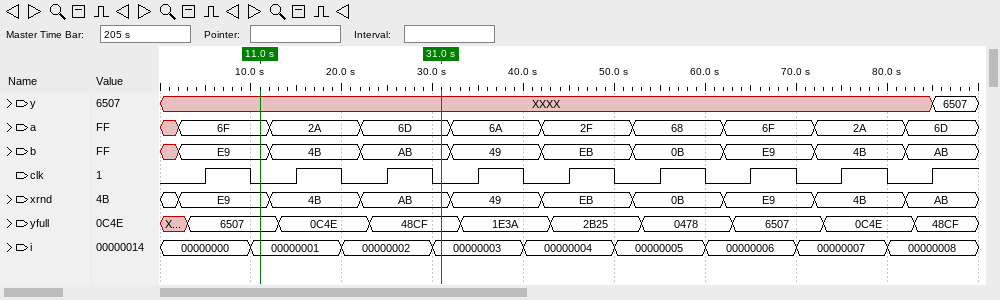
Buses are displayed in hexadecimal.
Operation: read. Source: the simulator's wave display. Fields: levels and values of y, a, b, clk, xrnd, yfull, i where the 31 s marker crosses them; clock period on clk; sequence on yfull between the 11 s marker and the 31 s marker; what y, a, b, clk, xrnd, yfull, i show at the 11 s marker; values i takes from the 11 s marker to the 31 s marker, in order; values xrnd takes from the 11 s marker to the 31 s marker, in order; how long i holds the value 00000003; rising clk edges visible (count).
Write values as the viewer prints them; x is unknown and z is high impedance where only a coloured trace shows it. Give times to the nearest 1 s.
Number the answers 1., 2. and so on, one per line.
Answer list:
1. y=XXXX, a=6D, b=AB, clk=0, xrnd=AB, yfull=48CF, i=00000003
2. 10 s
3. 6507, 0C4E, 48CF
4. y=XXXX, a=6F, b=E9, clk=0, xrnd=E9, yfull=6507, i=00000001
5. 00000001, 00000002, 00000003
6. E9, 4B, AB
7. 10 s
8. 9
